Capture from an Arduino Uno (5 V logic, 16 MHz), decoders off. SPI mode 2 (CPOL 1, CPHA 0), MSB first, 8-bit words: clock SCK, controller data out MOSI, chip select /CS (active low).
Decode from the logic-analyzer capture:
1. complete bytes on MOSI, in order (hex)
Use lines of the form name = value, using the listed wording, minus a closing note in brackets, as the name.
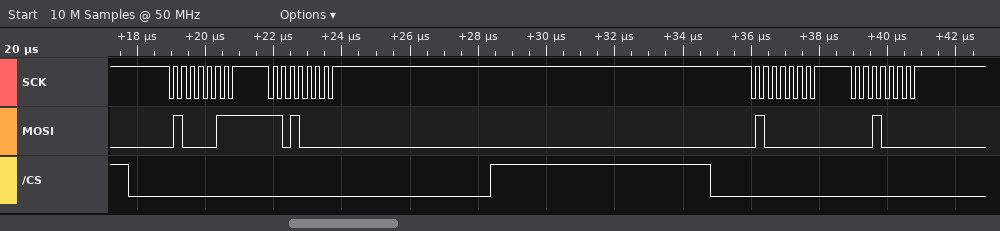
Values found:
complete bytes on MOSI, in order = 0x43 0xD0 0x40 0x10
